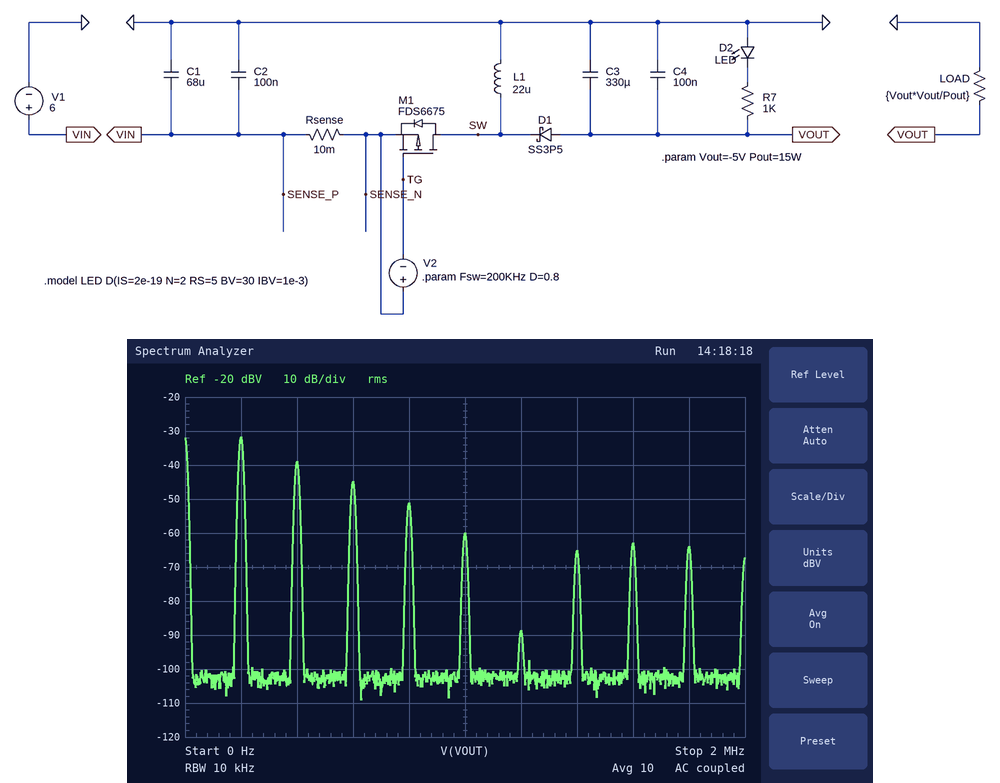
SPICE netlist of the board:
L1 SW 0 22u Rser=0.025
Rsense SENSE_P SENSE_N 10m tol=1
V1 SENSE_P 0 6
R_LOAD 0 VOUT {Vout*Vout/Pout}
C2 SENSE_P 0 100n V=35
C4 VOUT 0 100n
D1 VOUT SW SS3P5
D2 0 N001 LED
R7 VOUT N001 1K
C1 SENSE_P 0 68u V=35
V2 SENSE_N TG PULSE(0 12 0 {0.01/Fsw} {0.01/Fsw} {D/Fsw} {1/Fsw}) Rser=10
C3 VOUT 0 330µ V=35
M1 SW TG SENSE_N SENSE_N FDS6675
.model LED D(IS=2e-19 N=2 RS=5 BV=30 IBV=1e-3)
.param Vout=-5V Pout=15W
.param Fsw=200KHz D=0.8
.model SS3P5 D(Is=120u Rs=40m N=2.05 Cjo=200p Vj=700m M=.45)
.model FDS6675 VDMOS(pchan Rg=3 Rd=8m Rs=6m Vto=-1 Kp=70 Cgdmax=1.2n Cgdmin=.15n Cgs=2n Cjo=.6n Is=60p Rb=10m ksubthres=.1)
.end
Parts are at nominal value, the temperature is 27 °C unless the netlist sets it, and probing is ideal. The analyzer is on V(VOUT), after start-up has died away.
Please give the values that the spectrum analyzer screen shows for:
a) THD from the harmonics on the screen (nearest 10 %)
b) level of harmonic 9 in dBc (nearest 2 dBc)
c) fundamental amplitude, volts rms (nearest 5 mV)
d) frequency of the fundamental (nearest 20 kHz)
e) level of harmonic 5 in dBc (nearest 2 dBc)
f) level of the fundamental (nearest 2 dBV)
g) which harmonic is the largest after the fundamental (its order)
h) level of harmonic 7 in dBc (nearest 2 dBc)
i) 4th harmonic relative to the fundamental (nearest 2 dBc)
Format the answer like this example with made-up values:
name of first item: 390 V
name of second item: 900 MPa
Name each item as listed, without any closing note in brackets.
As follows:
THD from the harmonics on the screen: 50 %
level of harmonic 9 in dBc: -32 dBc
fundamental amplitude, volts rms: 25 mV
frequency of the fundamental: 200 kHz
level of harmonic 5 in dBc: -28 dBc
level of the fundamental: -32 dBV
which harmonic is the largest after the fundamental: 2
level of harmonic 7 in dBc: -34 dBc
4th harmonic relative to the fundamental: -20 dBc
